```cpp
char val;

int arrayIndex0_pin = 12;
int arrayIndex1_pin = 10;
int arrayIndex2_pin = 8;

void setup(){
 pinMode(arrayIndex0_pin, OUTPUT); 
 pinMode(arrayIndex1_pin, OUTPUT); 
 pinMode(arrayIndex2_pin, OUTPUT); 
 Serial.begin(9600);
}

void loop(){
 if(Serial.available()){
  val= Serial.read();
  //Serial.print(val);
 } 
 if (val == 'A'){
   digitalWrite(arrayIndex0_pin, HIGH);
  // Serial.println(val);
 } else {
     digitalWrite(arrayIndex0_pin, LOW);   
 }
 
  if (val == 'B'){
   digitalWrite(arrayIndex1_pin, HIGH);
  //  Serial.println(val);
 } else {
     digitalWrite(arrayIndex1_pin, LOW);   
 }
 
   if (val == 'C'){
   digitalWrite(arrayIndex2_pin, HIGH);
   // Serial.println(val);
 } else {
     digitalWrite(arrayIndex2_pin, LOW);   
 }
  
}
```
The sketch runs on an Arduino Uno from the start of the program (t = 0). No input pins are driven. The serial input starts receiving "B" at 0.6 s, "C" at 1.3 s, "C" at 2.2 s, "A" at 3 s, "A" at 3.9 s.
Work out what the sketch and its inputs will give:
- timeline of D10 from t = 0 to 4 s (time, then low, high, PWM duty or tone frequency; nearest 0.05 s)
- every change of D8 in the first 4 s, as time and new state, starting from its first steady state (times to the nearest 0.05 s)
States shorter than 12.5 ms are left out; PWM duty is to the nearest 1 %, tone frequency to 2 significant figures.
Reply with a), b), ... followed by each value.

a) 0 s low; 0.6 s high; 1.3 s low
b) 0 s low; 1.3 s high; 3 s low
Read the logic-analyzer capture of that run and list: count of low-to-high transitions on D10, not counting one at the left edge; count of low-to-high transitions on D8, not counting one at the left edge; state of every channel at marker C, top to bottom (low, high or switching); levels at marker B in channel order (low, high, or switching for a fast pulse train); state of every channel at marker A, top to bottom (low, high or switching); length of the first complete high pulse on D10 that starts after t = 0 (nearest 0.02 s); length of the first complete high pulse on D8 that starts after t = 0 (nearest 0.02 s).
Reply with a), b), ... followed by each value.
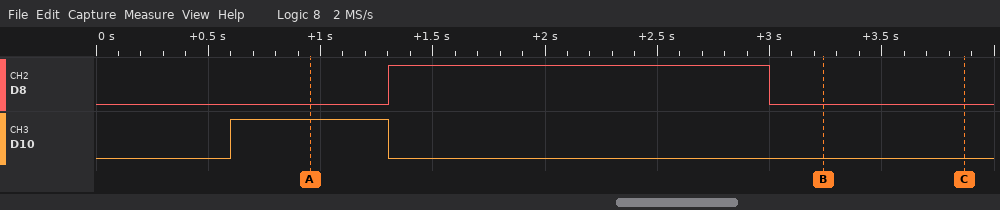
a) 1
b) 1
c) D8 low, D10 low
d) D8 low, D10 low
e) D8 low, D10 high
f) 0.70 s
g) 1.70 s
